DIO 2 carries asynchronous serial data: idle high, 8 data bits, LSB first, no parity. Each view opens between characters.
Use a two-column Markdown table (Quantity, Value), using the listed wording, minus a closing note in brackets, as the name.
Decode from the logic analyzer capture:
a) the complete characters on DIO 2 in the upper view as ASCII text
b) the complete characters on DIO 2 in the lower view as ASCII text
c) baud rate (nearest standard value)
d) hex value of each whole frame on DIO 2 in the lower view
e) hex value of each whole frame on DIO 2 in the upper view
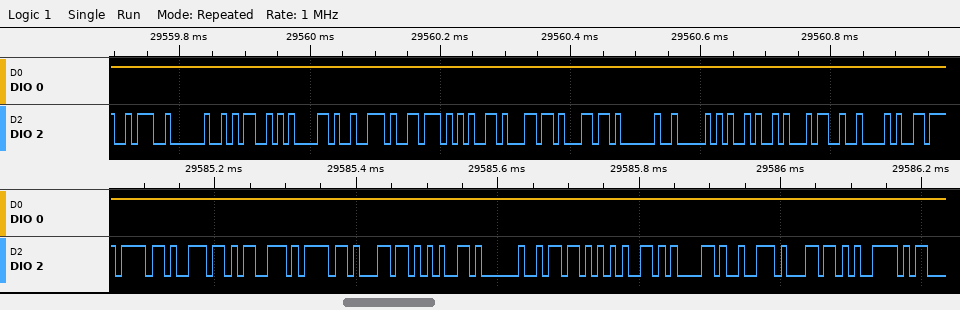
| Quantity | Value |
|---|---|
| the complete characters on DIO 2 in the upper view as ASCII text | ": Marvell PJ4B" |
| the complete characters on DIO 2 in the lower view as ASCII text | "onsole [early" |
| baud rate | 115200 baud |
| hex value of each whole frame on DIO 2 in the lower view | 6F, 6E, 73, 6F, 6C, 65, 20, 5B, 65, 61, 72, 6C, 79 |
| hex value of each whole frame on DIO 2 in the upper view | 3A, 20, 4D, 61, 72, 76, 65, 6C, 6C, 20, 50, 4A, 34, 42 |
